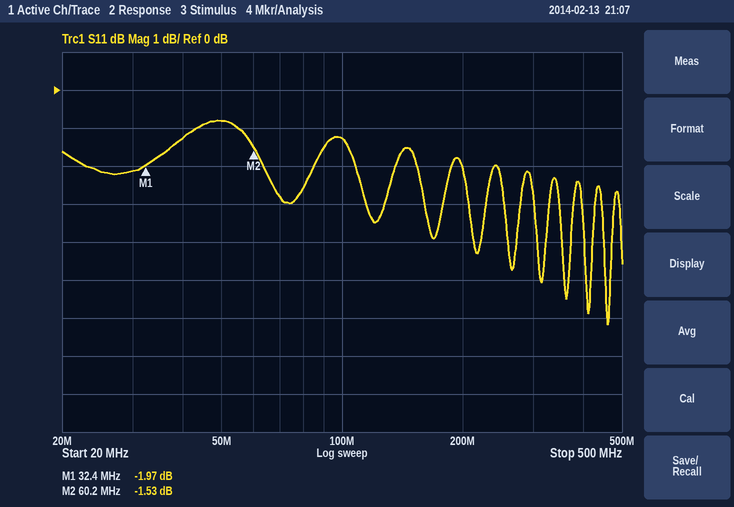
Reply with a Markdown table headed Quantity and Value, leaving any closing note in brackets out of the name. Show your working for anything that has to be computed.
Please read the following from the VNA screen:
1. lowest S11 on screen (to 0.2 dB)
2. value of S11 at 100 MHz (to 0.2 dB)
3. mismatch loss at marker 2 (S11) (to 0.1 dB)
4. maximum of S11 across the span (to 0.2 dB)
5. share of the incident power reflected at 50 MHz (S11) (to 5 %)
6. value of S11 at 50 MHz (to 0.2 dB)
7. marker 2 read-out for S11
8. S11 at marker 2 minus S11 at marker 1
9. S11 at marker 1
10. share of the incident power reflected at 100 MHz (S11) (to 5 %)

| Quantity | Value |
|---|---|
| lowest S11 on screen | -6.2 dB |
| value of S11 at 100 MHz | -1.2 dB |
| mismatch loss at marker 2 (S11) | −10 log10(1 − 10^(-1.53/10)) ≈ 5.3 dB |
| maximum of S11 across the span | -0.8 dB |
| share of the incident power reflected at 50 MHz (S11) | 10^(-0.8/10) ≈ 83.2 %, so 85 % to the nearest 5 % |
| value of S11 at 50 MHz | -0.8 dB |
| marker 2 read-out for S11 | -1.53 dB |
| S11 at marker 2 minus S11 at marker 1 | -1.53 − (-1.97) = 0.44 dB |
| S11 at marker 1 | -1.97 dB |
| share of the incident power reflected at 100 MHz (S11) | 10^(-1.2/10) ≈ 75.9 %, so 75 % to the nearest 5 % |
